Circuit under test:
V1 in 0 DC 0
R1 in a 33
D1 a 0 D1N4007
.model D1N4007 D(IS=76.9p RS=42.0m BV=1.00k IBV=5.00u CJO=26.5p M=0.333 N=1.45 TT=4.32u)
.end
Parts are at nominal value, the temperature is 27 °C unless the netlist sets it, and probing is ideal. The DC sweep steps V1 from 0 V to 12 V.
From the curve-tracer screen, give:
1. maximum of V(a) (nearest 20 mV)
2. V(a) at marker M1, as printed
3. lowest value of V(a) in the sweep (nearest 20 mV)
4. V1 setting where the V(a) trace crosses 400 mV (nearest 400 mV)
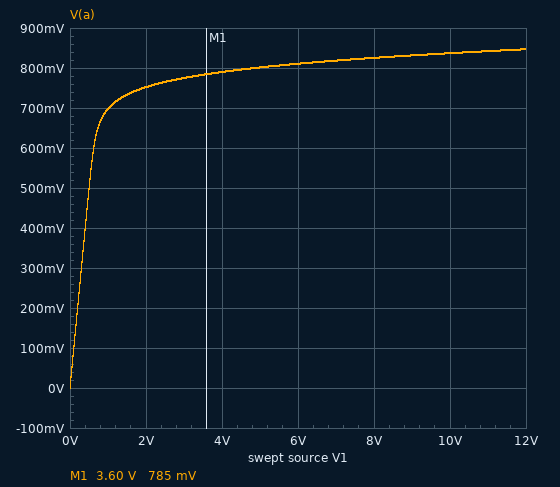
840 mV
785 mV
0 V
400 mV
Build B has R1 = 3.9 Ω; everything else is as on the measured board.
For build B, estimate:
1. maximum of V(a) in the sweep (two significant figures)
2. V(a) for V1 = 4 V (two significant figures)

1.0 V
900 mV
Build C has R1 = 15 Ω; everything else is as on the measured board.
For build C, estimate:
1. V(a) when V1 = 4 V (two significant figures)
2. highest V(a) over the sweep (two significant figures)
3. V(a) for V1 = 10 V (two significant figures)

820 mV
890 mV
880 mV
